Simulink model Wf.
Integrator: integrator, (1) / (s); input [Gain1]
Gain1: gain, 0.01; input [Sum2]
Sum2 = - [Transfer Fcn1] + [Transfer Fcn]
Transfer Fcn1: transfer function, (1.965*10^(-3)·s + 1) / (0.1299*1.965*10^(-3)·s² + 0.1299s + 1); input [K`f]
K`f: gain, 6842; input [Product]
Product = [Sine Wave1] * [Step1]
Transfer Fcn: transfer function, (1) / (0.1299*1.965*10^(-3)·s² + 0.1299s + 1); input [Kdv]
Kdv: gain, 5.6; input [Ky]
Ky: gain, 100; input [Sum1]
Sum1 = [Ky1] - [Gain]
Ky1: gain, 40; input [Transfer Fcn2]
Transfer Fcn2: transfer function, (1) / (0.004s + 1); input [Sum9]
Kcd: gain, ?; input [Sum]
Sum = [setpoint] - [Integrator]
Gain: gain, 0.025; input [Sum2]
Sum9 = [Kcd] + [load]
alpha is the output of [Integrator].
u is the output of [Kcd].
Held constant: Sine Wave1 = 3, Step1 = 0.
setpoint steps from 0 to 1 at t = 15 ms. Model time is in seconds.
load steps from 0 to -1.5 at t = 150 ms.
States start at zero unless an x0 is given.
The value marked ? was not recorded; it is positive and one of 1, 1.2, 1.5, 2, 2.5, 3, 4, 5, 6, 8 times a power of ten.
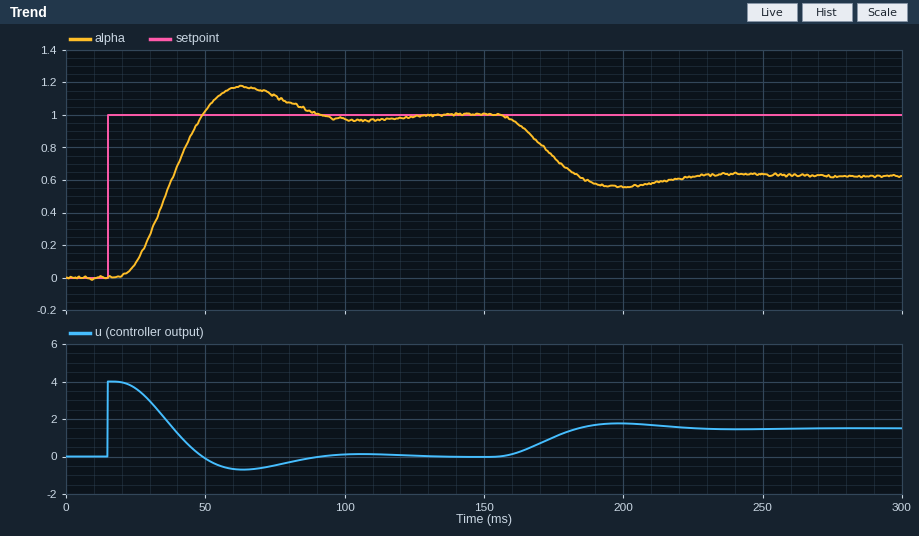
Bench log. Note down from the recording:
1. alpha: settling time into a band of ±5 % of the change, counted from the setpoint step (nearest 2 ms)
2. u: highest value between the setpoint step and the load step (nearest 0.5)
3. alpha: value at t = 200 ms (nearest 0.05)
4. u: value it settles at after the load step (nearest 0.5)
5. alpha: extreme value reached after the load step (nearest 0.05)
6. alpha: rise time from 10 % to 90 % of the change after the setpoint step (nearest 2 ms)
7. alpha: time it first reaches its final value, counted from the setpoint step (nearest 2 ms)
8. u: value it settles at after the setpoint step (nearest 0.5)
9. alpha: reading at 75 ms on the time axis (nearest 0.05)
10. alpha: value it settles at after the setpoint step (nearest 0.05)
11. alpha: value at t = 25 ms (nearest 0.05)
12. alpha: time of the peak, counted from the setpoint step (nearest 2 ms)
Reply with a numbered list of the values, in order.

1. 68 ms
2. 4.0
3. 0.55
4. 1.5
5. 0.55
6. 20 ms
7. 34 ms
8. 0.0
9. 1.10
10. 1.00
11. 0.10
12. 48 ms
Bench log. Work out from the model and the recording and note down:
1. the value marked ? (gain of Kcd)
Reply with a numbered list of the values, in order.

1. 4
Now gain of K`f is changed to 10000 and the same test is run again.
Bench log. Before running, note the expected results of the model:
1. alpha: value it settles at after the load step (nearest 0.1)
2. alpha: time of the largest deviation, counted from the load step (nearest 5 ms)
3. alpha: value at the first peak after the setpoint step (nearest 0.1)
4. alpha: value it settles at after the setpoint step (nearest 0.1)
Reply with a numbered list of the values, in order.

1. 0.6
2. 50 ms
3. 1.2
4. 1.0
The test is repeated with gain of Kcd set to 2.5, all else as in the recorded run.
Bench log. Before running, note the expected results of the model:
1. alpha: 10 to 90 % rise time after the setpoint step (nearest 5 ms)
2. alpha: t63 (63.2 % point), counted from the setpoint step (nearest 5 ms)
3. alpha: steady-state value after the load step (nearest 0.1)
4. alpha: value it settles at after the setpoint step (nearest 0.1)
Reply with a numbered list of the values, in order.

1. 35 ms
2. 30 ms
3. 0.4
4. 1.0
